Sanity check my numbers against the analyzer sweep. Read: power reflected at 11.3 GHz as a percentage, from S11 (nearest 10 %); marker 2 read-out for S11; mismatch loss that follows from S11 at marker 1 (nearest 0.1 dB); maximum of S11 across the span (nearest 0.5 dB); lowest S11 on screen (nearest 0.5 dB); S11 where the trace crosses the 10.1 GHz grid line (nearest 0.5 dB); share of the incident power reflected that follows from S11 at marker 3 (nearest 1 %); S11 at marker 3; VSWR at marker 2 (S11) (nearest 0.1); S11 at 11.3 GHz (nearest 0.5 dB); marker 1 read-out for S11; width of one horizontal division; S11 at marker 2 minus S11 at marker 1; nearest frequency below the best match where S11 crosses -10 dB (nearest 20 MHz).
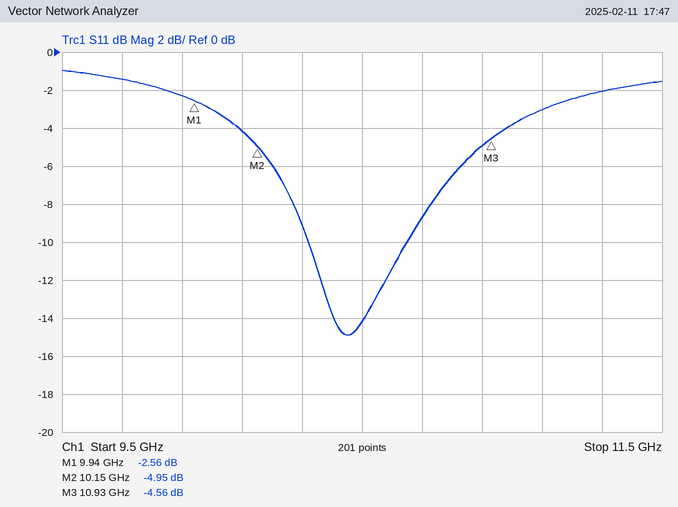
60 %
-4.95 dB
3.5 dB
-1.0 dB
-15.0 dB
-4.0 dB
35 %
-4.56 dB
3.6
-2.0 dB
-2.56 dB
200 MHz
-2.39 dB
10.32 GHz
